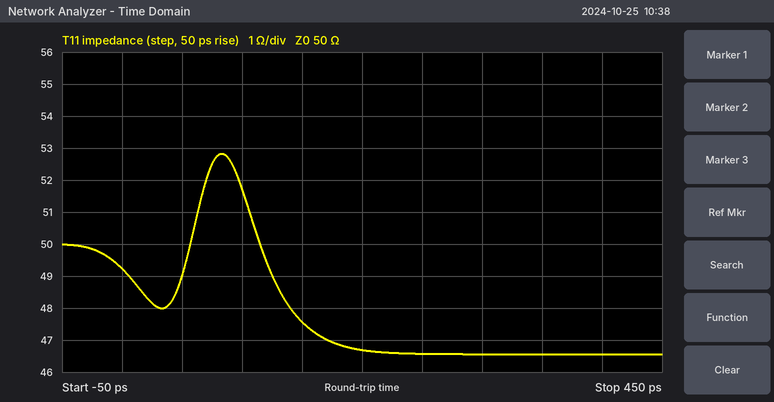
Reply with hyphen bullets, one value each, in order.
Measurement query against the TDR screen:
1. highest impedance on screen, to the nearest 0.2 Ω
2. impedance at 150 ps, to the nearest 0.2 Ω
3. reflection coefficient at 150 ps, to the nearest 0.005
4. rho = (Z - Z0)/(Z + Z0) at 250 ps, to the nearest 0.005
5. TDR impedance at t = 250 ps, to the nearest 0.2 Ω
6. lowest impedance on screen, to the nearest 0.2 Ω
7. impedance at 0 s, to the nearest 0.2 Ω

- 52.8 Ω
- 47.6 Ω
- -0.025
- -0.035
- 46.6 Ω
- 46.6 Ω
- 49.2 Ω
